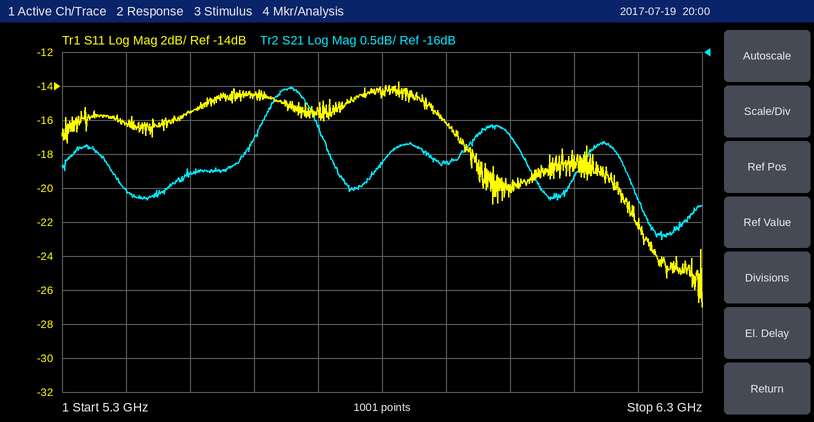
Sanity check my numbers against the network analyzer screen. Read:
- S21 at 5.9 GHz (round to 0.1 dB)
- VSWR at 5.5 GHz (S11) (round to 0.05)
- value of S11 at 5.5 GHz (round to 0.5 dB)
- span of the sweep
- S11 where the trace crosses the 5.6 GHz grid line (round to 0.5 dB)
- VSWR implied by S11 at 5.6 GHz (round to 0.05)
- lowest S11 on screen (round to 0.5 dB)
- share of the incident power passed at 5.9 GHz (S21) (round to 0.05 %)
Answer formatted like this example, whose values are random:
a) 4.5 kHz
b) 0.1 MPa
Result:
a) -17.6 dB
b) 1.40
c) -15.5 dB
d) 1 GHz
e) -14.5 dB
f) 1.45
g) -27.0 dB
h) 1.75 %
